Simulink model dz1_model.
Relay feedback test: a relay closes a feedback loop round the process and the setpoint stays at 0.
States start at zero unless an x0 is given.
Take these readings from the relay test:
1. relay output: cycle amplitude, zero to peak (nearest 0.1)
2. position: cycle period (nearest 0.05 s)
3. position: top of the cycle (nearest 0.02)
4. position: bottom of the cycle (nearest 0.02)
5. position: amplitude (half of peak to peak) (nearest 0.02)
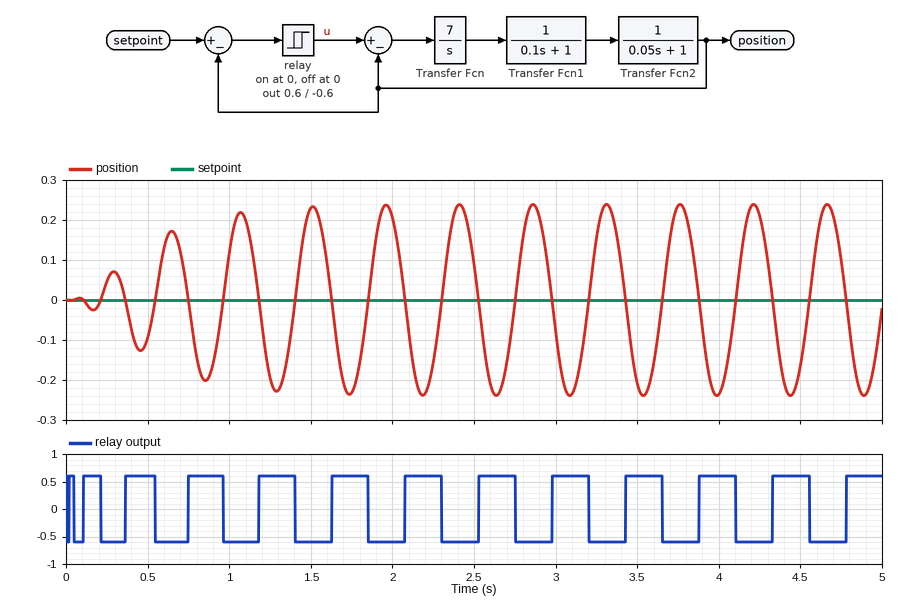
0.6
0.45 s
0.24
-0.24
0.24
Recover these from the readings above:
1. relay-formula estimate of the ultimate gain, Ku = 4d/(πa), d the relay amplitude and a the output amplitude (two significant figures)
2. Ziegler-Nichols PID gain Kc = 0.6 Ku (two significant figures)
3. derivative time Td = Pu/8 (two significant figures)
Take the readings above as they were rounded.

3.2
1.9
0.056 s
